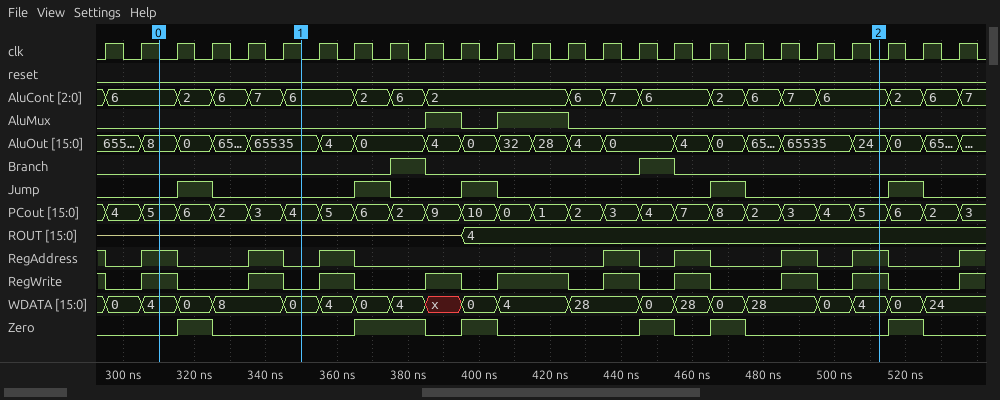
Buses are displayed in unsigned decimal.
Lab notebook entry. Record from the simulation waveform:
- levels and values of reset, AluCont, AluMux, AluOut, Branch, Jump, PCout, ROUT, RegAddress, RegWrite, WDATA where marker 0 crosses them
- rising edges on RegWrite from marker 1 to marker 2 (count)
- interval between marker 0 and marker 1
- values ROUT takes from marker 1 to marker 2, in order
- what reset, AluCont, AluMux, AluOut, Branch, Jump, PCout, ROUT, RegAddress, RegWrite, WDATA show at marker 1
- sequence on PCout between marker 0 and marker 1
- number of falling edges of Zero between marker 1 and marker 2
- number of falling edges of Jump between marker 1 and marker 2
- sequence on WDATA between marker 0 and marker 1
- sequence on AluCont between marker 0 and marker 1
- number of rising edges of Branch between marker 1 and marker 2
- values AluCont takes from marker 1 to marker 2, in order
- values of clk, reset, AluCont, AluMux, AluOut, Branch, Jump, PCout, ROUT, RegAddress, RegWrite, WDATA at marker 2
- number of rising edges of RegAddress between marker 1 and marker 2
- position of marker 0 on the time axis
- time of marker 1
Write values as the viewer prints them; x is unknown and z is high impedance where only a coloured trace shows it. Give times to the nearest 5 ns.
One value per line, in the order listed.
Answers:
reset=0, AluCont=6, AluMux=0, AluOut=8, Branch=0, Jump=0, PCout=5, ROUT=z, RegAddress=1, RegWrite=1, WDATA=4
7
40 ns
z, 4
reset=0, AluCont=6, AluMux=0, AluOut=65535, Branch=0, Jump=0, PCout=4, ROUT=z, RegAddress=0, RegWrite=0, WDATA=0
5, 6, 2, 3, 4
4
3
4, 0, 8, 0
6, 2, 6, 7, 6
2
6, 2, 6, 2, 6, 7, 6, 2, 6, 7, 6
clk=0, reset=0, AluCont=6, AluMux=0, AluOut=24, Branch=0, Jump=0, PCout=5, ROUT=4, RegAddress=1, RegWrite=1, WDATA=4
5
310 ns
350 ns
